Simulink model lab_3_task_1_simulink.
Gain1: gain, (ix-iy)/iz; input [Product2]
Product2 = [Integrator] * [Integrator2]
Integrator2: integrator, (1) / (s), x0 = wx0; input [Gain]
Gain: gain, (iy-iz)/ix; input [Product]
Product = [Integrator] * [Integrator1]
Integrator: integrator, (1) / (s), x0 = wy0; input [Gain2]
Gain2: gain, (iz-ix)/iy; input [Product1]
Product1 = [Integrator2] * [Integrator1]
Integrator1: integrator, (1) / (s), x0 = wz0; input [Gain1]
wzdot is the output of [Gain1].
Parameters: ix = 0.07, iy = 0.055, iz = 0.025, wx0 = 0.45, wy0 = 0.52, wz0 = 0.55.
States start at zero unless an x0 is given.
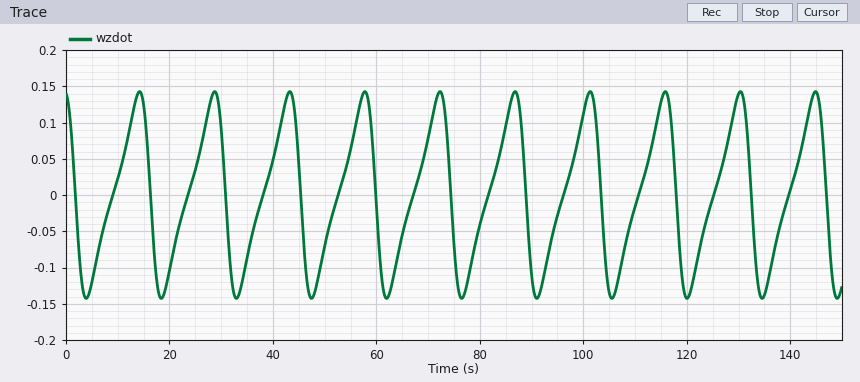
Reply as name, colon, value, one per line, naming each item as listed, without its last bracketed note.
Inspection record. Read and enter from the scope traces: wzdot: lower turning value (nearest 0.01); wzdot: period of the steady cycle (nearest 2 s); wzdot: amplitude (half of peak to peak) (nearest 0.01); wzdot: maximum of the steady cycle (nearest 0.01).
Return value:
wzdot: lower turning value: -0.14
wzdot: period of the steady cycle: 14 s
wzdot: amplitude (half of peak to peak): 0.14
wzdot: maximum of the steady cycle: 0.14
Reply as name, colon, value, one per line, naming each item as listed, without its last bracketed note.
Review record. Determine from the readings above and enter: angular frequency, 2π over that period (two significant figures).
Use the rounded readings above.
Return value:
angular frequency, 2π over that period: 0.45 rad/s
